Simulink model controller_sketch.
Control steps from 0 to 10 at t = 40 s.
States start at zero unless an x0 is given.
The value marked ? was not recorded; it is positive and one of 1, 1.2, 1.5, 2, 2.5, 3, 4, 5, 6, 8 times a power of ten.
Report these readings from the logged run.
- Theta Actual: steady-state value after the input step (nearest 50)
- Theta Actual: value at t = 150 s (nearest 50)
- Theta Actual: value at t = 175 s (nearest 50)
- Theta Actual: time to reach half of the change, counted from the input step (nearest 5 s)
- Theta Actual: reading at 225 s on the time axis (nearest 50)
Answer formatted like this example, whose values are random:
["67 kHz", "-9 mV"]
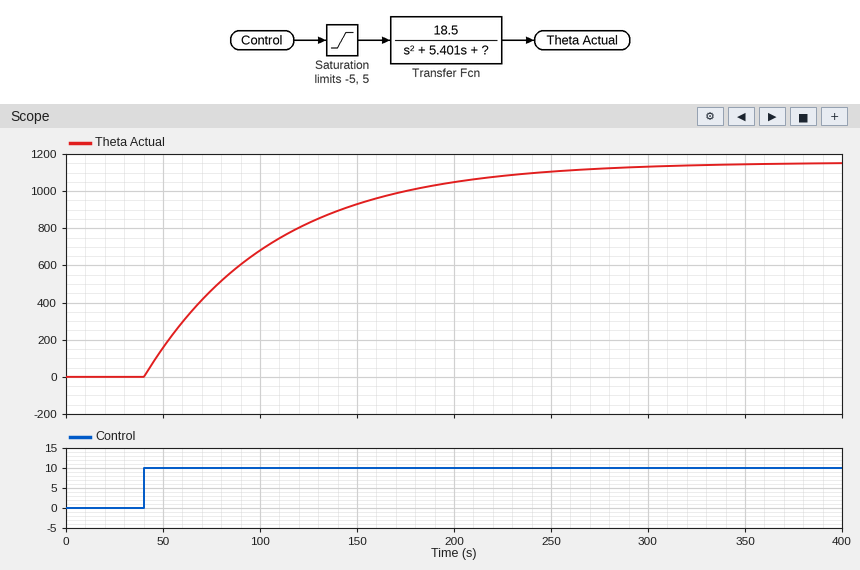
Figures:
["1150", "950", "1000", "45 s", "1100"]
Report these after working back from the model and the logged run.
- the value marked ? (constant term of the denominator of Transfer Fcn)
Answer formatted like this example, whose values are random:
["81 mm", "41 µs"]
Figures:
["0.08"]
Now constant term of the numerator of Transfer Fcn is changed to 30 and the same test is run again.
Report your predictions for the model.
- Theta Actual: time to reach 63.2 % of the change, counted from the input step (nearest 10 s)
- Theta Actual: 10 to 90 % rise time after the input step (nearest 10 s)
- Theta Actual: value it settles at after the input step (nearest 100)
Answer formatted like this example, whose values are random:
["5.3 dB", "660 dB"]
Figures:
["70 s", "150 s", "1900"]
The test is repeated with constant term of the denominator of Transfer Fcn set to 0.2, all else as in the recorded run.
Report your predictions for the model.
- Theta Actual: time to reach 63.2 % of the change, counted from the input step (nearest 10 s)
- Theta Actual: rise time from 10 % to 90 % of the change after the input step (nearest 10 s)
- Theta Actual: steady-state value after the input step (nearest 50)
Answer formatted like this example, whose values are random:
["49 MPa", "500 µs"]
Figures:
["30 s", "60 s", "450"]
